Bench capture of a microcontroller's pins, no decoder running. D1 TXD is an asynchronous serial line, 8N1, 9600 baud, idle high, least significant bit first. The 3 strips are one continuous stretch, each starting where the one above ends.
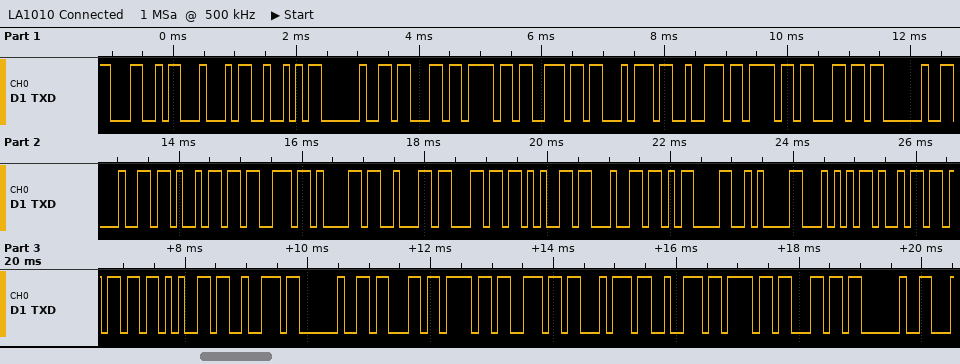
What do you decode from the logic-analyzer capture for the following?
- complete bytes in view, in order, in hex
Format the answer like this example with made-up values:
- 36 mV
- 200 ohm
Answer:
- 0x4C 0x44 0x52 0x20 0x63 0x6F 0x6E 0x74 0x72 0x6F 0x6C 0x20 0x64 0x69 0x73 0x61 0x62 0x6C 0x65 0x64 0x0D 0x0A 0x54 0x69 0x6D 0x65 0x72 0x20 0x63 0x6F 0x6E 0x74 0x72 0x6F 0x6C 0x20
